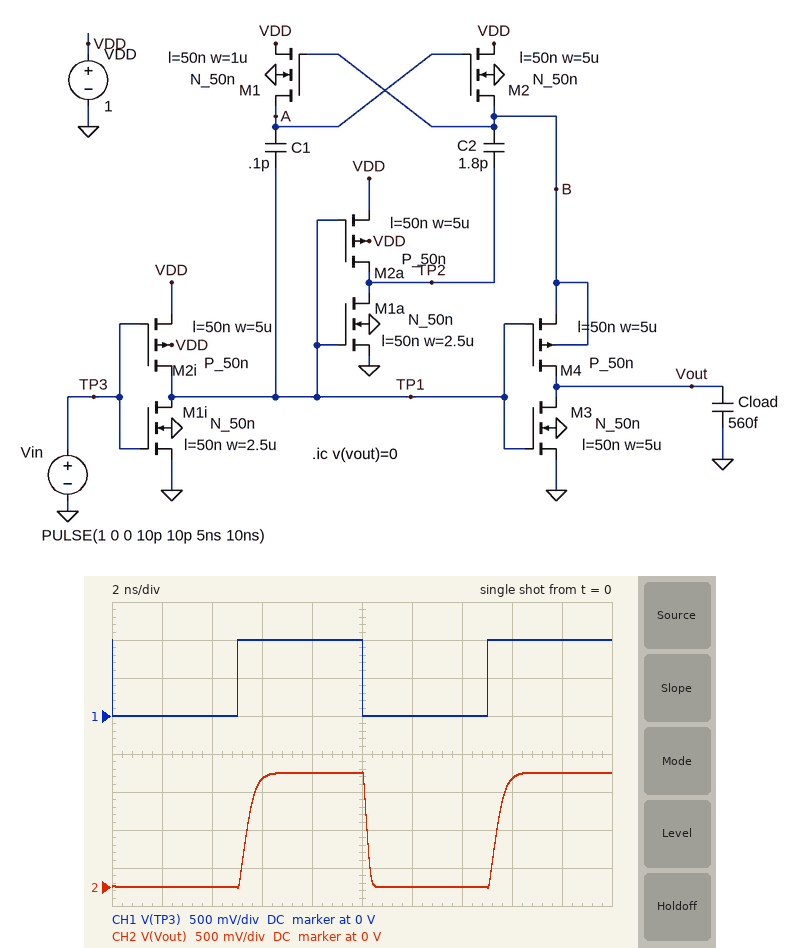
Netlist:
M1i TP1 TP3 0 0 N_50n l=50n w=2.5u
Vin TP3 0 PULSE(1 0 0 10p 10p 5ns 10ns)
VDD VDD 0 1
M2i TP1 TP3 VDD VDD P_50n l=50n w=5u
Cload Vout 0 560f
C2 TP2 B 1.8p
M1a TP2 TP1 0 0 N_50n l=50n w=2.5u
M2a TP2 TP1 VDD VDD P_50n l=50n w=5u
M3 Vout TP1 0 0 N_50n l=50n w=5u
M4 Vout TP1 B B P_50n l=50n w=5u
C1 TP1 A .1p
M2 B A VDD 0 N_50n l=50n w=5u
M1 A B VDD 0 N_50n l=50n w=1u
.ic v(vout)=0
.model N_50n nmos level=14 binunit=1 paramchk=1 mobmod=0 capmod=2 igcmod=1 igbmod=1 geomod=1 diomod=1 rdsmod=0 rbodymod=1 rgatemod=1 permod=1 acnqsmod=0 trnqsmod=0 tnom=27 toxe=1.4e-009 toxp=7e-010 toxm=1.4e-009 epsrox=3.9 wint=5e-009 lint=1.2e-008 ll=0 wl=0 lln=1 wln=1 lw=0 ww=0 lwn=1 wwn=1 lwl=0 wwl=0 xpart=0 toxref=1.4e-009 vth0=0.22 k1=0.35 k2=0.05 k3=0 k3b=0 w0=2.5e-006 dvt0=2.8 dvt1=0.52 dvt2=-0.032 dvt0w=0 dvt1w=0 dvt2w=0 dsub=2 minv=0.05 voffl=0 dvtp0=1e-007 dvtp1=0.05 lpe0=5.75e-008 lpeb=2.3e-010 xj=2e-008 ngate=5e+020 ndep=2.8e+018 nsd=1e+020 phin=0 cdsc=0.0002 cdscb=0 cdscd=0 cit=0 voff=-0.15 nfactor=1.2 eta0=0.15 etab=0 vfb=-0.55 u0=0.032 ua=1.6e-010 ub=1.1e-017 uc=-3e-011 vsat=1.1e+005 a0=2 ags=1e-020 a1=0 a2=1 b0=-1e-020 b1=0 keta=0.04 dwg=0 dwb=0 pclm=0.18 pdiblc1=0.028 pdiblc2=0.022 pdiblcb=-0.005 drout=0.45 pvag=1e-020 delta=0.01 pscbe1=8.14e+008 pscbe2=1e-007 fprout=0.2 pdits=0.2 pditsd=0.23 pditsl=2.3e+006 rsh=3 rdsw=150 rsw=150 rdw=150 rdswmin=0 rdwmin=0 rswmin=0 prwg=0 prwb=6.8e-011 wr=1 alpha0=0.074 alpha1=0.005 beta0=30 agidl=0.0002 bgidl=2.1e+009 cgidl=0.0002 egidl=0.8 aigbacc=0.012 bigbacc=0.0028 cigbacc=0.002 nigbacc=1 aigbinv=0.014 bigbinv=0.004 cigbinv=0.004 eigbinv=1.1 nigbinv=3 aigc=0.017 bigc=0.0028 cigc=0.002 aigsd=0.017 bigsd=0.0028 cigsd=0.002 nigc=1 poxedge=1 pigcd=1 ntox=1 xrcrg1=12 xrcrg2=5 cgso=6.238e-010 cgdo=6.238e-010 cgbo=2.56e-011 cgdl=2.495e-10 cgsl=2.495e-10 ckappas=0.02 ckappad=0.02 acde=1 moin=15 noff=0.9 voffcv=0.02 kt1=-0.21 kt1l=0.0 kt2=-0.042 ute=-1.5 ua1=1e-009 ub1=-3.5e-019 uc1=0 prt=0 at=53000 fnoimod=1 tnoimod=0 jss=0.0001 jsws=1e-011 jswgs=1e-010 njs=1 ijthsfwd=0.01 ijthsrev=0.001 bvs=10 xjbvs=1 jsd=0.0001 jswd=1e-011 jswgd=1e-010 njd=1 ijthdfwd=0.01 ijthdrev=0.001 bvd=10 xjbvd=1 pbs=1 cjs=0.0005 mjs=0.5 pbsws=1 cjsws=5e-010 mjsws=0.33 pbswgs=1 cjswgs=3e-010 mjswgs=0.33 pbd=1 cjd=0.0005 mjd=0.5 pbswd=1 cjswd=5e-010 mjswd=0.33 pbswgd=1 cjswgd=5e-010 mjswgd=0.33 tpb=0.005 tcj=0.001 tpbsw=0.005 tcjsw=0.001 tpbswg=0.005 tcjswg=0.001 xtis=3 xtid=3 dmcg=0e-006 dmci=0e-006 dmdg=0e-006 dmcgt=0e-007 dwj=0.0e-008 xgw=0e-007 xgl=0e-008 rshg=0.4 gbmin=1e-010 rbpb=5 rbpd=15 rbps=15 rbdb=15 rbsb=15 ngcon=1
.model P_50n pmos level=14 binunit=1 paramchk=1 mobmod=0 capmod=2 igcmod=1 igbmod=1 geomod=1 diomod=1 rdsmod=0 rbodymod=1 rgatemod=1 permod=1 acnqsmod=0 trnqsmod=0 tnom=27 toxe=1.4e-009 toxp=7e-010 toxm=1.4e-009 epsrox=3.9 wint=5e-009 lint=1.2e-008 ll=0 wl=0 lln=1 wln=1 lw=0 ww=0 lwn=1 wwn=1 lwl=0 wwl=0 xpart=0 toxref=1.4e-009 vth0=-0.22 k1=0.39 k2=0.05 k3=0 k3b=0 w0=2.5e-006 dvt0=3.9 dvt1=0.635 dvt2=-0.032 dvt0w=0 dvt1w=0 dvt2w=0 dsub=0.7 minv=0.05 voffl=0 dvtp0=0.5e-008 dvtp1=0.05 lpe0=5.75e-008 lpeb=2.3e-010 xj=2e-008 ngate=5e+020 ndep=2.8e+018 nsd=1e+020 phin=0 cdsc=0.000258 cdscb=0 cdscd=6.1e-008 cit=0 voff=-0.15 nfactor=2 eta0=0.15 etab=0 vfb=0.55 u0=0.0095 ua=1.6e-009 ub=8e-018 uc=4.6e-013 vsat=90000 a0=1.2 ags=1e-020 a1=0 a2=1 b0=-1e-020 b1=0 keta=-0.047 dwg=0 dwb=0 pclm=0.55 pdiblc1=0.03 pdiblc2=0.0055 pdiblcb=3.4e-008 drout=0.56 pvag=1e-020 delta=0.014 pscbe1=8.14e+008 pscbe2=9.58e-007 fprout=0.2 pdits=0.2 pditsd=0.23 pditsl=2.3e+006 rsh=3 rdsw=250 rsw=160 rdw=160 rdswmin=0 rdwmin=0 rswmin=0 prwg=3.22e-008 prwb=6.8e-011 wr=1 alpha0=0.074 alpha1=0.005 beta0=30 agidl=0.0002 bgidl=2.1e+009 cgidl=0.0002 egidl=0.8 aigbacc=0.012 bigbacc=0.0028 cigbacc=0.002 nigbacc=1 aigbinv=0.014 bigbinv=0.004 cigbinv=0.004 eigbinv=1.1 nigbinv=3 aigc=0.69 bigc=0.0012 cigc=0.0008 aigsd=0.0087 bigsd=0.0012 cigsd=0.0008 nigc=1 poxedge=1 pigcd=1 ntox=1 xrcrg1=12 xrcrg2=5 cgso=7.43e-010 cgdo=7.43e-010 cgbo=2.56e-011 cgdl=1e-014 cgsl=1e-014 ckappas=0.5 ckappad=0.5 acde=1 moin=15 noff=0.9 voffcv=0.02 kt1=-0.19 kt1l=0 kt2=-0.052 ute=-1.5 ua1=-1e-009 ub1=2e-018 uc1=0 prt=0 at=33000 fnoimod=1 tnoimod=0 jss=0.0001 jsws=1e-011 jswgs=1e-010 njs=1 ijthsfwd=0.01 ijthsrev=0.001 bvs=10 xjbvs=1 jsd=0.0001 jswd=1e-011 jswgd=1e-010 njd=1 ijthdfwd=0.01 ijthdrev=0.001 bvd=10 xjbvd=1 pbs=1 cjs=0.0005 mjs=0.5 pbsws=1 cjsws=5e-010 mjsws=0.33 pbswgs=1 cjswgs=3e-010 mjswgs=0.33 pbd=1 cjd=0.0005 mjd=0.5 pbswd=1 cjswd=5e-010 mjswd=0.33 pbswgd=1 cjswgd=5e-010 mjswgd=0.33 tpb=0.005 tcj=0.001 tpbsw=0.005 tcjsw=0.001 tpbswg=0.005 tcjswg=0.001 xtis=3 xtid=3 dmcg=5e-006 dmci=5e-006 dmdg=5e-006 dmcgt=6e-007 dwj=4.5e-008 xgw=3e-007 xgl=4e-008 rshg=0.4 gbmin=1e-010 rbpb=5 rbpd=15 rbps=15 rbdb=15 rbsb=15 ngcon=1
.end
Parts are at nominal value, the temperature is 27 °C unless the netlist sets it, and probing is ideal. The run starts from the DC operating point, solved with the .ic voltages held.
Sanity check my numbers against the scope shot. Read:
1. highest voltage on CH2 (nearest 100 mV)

1.5 V
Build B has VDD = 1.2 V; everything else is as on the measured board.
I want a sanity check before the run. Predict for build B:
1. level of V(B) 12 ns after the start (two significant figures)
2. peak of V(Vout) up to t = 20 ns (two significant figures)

1.2 V
1.8 V
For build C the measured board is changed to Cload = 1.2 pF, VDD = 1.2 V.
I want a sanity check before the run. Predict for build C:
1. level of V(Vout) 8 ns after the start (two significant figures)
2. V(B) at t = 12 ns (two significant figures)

1.4 V
1.2 V
